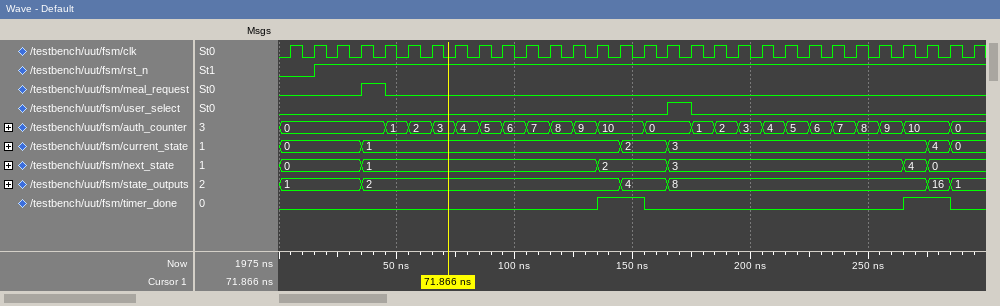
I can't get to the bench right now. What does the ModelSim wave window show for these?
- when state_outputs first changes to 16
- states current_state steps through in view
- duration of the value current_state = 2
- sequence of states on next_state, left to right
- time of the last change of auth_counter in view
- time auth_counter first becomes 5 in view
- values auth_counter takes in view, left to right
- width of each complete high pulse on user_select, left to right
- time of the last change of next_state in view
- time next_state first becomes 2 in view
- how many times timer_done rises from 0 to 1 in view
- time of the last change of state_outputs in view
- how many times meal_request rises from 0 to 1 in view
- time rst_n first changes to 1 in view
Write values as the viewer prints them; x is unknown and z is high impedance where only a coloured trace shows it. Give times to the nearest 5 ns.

275 ns
0, 1, 2, 3, 4, 0
20 ns
0, 1, 2, 3, 4, 0
285 ns
85 ns
0, 1, 2, 3, 4, 5, 6, 7, 8, 9, 10, 0, 1, 2, 3, 4, 5, 6, 7, 8, 9, 10, 0
10 ns
275 ns
135 ns
2
285 ns
1
15 ns
